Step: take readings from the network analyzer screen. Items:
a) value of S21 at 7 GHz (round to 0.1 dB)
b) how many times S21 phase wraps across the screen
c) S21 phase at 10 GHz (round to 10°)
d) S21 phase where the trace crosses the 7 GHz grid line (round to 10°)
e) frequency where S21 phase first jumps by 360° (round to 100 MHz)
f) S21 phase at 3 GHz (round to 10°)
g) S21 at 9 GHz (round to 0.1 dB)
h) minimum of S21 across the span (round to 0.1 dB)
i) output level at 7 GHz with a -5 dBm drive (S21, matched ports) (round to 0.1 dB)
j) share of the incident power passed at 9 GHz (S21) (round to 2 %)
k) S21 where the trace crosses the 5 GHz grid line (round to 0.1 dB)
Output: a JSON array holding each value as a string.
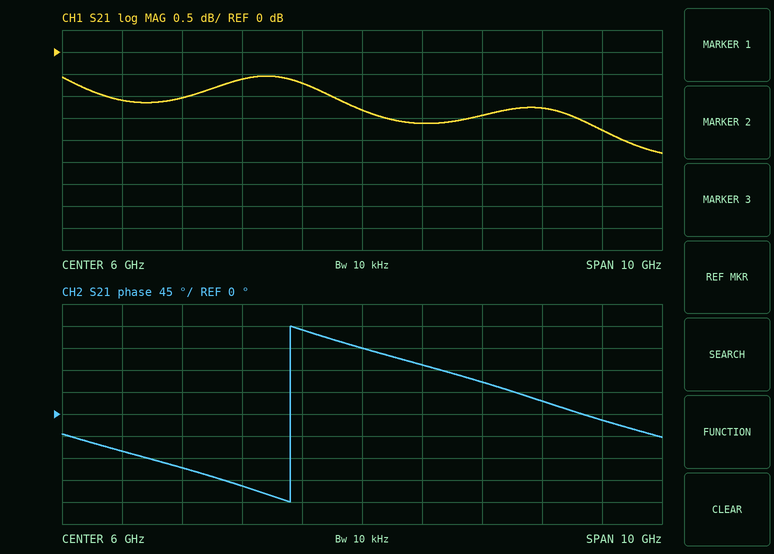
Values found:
["-1.6 dB", "1", "-10°", "100°", "4.8 GHz", "-110°", "-1.3 dB", "-2.3 dB", "-6.6 dBm", "74 %", "-0.7 dB"]
